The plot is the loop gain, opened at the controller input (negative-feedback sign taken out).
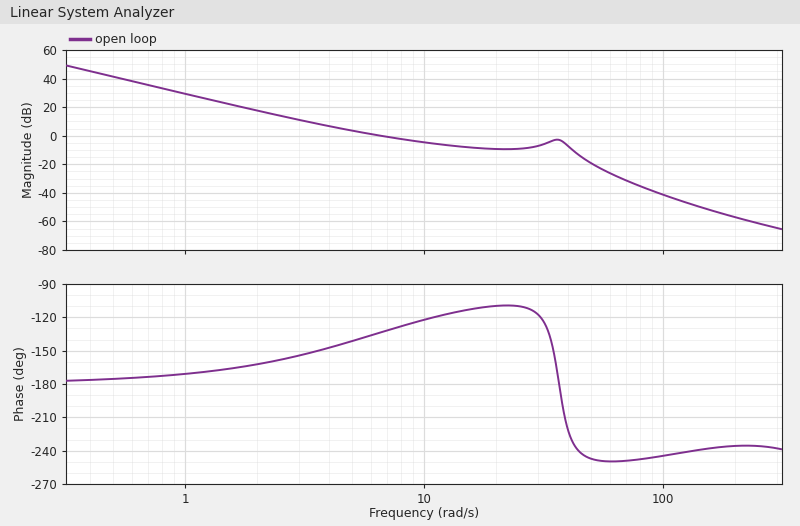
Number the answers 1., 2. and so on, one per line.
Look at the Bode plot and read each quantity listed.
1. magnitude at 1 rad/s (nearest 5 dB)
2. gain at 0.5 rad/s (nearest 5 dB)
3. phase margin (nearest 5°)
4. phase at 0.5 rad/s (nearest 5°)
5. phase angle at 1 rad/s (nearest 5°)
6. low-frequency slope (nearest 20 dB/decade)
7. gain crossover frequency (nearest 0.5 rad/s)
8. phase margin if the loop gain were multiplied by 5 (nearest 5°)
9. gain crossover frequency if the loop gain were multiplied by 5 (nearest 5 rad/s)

1. 30 dB
2. 40 dB
3. 45°
4. -175°
5. -170°
6. -40 dB/decade
7. 6.5 rad/s
8. -60°
9. 45 rad/s
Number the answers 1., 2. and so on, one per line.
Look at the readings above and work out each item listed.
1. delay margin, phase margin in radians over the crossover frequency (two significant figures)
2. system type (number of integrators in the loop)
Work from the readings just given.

1. 0.12 s
2. 2
